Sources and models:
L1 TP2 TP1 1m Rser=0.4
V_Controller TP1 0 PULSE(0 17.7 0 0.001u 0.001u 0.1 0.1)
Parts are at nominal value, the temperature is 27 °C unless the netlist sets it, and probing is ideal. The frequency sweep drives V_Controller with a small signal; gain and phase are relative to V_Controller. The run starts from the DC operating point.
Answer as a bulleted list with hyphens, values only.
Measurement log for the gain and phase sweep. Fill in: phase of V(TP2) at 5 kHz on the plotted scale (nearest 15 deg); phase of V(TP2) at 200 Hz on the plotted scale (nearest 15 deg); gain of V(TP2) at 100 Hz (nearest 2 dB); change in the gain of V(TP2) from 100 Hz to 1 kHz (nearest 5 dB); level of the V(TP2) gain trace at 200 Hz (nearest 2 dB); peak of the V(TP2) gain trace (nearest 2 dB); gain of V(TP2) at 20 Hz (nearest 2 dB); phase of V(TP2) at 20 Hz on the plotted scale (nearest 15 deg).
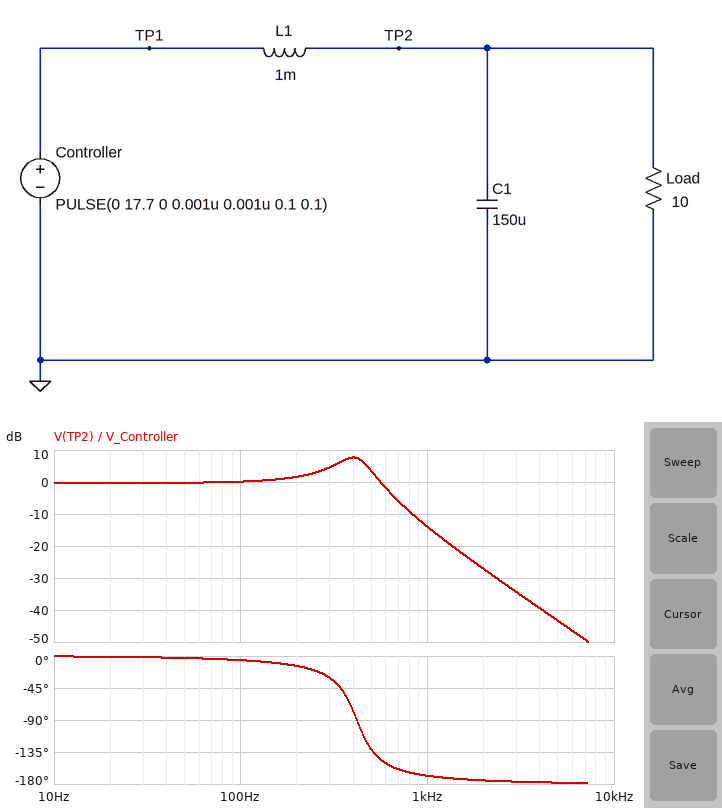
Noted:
- -180 deg
- -15 deg
- 0 dB
- -15 dB
- 2 dB
- 8 dB
- 0 dB
- 0 deg
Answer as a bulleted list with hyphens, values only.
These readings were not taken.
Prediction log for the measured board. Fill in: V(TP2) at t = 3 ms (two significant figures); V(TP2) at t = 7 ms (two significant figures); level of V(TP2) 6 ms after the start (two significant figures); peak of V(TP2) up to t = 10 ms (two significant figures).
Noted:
- 16 V
- 17 V
- 18 V
- 26 V
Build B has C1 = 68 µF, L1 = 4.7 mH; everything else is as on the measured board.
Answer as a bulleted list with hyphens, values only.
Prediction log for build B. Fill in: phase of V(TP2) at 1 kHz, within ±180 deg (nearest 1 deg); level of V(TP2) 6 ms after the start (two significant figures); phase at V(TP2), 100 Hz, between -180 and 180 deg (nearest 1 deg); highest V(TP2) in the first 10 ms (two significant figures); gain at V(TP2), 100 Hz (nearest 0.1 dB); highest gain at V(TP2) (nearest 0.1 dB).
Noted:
- -165 deg
- 17 V
- -19 deg
- 21 V
- 0.3 dB
- 1.8 dB
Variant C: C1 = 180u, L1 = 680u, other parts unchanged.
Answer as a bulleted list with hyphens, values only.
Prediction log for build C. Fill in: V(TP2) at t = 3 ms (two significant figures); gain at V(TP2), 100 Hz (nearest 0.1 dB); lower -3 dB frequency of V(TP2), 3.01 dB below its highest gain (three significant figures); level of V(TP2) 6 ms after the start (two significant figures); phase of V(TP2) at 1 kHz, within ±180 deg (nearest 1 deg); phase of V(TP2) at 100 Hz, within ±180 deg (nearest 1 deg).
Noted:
- 19 V
- 0 dB
- 340 Hz
- 17 V
- -167 deg
- -5 deg
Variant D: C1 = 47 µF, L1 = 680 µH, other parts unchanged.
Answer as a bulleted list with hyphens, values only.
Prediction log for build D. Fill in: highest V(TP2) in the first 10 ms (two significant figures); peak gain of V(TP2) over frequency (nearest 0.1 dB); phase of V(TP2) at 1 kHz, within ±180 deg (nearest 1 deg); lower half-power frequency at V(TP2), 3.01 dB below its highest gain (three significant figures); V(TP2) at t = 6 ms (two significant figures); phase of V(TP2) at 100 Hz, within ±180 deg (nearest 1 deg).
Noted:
- 25 V
- 6.4 dB
- -112 deg
- 591 Hz
- 17 V
- -3 deg
